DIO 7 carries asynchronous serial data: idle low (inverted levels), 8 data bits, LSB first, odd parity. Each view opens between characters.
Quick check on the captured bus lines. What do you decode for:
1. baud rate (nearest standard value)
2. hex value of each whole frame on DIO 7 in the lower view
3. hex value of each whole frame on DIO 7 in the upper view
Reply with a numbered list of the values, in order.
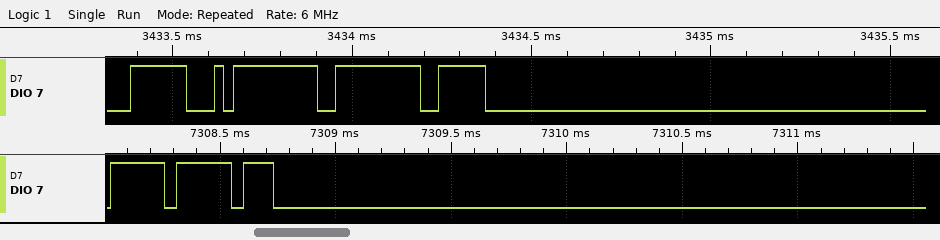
1. 38400 baud
2. 00, 00, F0
3. E0, 00, 00, F0
